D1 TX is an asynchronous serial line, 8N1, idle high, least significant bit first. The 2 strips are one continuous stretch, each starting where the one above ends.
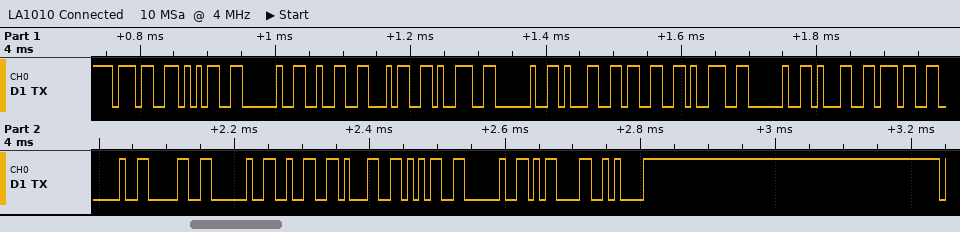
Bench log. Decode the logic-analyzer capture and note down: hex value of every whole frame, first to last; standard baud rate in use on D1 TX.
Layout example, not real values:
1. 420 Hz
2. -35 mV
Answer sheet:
1. 37 35 20 32 34 39 20 31 33 39 20 31 37 20 30 20 32 31 35 20 0D 0A
2. 115200 baud
